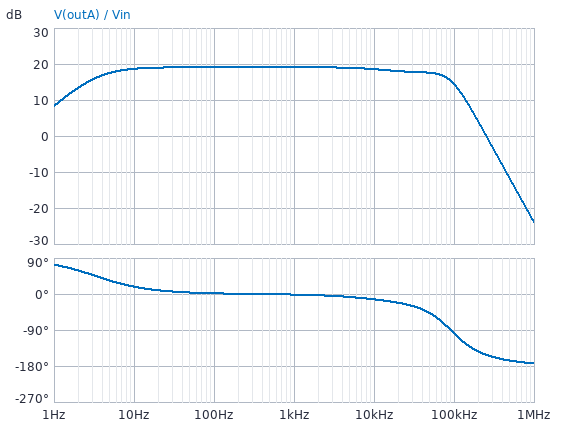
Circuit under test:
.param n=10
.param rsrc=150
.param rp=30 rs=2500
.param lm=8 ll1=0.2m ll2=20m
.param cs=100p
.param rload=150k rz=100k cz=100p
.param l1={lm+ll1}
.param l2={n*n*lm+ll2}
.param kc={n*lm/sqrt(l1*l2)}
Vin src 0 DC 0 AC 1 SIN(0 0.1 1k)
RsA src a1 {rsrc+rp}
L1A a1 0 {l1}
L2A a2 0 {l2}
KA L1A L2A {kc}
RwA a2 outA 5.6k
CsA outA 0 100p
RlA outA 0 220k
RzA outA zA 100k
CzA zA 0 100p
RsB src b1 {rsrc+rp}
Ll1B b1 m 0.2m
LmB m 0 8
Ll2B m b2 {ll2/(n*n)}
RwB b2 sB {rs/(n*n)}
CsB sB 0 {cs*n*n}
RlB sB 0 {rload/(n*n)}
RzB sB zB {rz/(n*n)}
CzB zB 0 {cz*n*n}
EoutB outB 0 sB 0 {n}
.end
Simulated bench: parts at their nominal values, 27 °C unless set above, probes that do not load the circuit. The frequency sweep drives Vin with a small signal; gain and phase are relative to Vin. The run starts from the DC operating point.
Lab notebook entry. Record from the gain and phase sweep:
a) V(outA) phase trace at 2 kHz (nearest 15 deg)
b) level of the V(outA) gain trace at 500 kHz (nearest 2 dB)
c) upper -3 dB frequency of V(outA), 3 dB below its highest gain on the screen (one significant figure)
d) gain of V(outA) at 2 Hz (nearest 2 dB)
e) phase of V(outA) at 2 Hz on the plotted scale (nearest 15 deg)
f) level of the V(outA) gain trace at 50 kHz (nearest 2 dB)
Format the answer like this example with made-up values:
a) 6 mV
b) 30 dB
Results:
a) 0 deg
b) -12 dB
c) 80 kHz
d) 14 dB
e) 60 deg
f) 18 dB
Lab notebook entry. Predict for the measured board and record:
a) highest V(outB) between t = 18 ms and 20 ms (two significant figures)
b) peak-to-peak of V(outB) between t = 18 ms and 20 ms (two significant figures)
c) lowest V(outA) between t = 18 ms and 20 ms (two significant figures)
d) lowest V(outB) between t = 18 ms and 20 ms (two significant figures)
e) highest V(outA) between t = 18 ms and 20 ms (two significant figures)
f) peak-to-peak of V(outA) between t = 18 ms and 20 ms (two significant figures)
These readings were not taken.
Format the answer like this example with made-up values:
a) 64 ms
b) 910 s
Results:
a) 880 mV
b) 1.8 V
c) -900 mV
d) -880 mV
e) 900 mV
f) 1.8 V
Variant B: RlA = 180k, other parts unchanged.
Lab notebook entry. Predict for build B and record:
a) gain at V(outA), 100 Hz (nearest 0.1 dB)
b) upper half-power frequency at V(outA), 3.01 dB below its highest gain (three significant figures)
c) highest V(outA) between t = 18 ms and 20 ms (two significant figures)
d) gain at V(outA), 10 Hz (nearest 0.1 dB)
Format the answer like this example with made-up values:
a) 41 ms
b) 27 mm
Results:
a) 18.9 dB
b) 82.4 kHz
c) 880 mV
d) 18.5 dB
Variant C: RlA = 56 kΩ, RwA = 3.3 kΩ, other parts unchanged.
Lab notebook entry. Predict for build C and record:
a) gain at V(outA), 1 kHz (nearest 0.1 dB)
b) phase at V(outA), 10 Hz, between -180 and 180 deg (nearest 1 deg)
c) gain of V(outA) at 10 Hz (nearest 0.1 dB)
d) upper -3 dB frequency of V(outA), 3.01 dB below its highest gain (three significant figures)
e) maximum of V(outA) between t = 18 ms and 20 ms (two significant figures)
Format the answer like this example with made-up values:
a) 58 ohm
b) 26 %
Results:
a) 17.2 dB
b) 15 deg
c) 16.9 dB
d) 94.1 kHz
e) 720 mV
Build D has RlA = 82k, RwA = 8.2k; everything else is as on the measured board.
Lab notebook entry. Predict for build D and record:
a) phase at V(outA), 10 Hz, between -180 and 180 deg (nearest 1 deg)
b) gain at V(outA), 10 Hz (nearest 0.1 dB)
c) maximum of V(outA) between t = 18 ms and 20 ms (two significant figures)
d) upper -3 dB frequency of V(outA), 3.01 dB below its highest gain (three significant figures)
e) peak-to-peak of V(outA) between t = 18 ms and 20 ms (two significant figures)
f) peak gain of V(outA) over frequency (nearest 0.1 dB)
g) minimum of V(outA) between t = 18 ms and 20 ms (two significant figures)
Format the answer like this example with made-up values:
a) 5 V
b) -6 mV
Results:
a) 17 deg
b) 17.2 dB
c) 760 mV
d) 79.0 kHz
e) 1.5 V
f) 17.6 dB
g) -760 mV
